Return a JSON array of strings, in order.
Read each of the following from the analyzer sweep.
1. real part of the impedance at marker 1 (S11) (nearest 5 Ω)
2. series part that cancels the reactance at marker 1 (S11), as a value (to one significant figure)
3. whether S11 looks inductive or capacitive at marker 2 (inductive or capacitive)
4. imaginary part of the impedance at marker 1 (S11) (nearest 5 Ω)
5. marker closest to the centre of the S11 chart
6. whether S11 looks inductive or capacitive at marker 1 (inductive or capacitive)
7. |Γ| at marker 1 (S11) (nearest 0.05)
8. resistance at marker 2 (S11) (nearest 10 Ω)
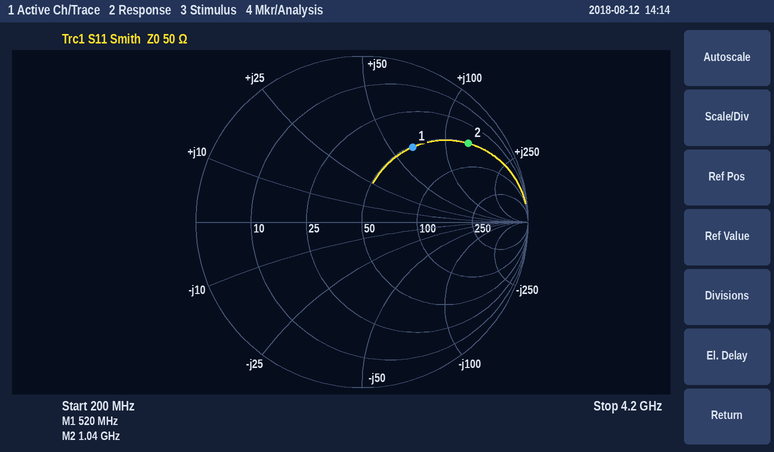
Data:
["50 Ω", "5 pF", "inductive", "+65 Ω", "marker 1", "inductive", "0.55", "50 Ω"]
